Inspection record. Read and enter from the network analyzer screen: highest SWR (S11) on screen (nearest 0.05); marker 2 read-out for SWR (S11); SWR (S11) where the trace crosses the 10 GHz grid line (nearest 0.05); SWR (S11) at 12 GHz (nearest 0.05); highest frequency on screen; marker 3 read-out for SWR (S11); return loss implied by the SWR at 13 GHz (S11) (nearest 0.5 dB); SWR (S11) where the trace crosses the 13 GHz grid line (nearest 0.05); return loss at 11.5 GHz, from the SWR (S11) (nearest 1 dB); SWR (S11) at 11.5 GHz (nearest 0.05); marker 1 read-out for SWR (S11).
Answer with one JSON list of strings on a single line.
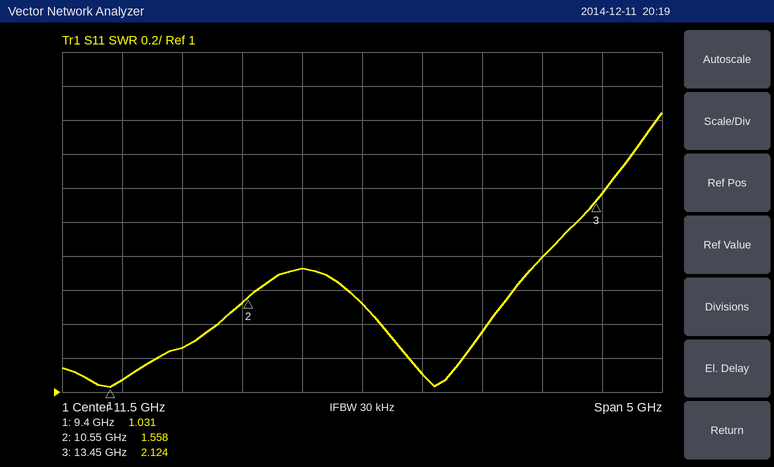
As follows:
["2.65", "1.558", "1.25", "1.10", "14 GHz", "2.124", "11.0 dB", "1.80", "14 dB", "1.50", "1.031"]
